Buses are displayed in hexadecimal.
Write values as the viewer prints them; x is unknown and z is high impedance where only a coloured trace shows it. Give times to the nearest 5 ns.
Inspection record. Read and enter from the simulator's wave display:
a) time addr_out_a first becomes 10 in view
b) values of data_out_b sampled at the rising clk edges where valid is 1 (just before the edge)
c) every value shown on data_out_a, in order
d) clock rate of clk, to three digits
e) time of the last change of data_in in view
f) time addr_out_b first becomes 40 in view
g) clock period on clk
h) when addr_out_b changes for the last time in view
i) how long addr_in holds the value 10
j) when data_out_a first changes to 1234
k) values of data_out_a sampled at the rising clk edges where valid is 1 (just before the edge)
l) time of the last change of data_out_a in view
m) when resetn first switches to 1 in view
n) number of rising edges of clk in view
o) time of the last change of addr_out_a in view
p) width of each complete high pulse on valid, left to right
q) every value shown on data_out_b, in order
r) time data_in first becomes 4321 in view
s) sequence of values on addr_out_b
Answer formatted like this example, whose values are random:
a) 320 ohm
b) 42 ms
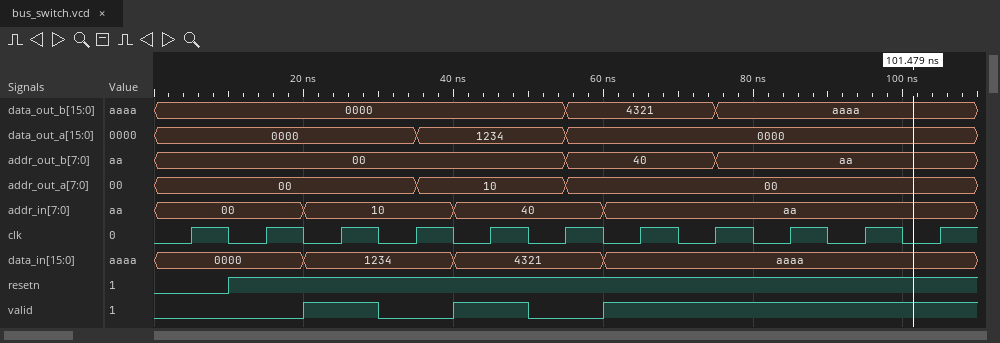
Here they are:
a) 35 ns
b) 0000, 0000, 4321, 4321, aaaa, aaaa, aaaa
c) 0000, 1234, 0000
d) 100 MHz
e) 60 ns
f) 55 ns
g) 10 ns
h) 75 ns
i) 20 ns
j) 35 ns
k) 0000, 1234, 0000, 0000, 0000, 0000, 0000
l) 55 ns
m) 10 ns
n) 11
o) 55 ns
p) 10 ns, 10 ns
q) 0000, 4321, aaaa
r) 40 ns
s) 00, 40, aa
